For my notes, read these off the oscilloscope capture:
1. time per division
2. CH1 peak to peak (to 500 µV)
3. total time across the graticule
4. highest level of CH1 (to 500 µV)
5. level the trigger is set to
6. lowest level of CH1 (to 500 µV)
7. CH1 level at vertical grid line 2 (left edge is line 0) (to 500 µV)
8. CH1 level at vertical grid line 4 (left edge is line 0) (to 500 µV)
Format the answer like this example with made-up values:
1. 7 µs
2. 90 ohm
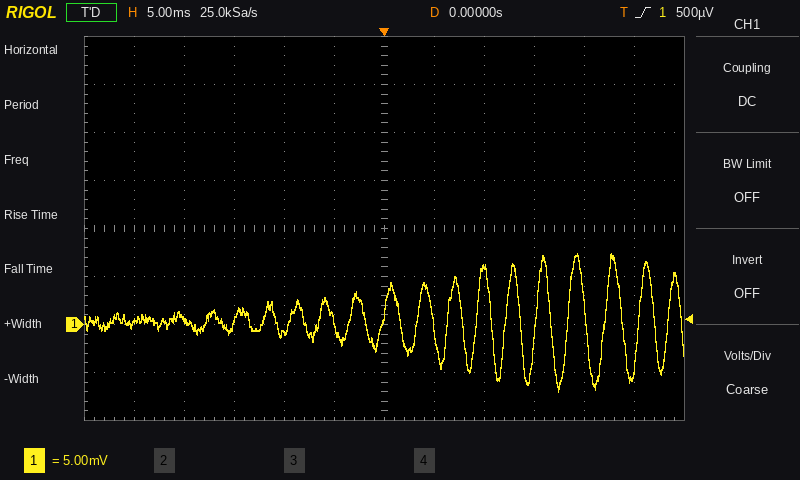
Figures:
1. 5 ms
2. 14.5 mV
3. 60 ms
4. 7.5 mV
5. 500 µV
6. -7.0 mV
7. 500 µV
8. -1.0 mV
